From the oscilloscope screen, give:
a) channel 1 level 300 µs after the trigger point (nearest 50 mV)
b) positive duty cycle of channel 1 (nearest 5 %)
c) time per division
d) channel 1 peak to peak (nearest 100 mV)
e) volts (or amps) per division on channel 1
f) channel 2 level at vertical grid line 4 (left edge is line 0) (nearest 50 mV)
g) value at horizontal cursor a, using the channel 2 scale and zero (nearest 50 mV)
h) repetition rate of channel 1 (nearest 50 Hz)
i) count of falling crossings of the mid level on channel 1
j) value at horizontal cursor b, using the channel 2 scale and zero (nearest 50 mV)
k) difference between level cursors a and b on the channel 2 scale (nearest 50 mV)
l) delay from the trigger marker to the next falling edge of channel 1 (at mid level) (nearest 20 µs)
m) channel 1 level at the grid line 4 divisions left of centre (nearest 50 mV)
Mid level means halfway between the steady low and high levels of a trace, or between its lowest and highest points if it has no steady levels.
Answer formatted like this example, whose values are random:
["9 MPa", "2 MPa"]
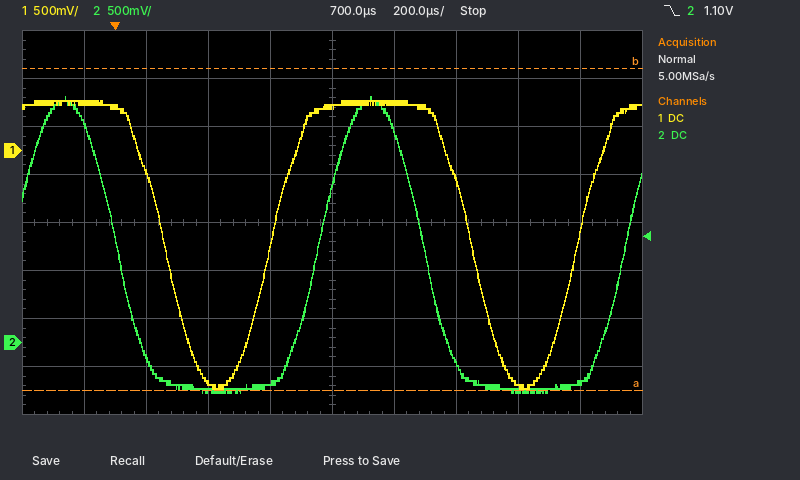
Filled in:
["-2.40 V", "65 %", "200 µs", "3.00 V", "500 mV", "-400 mV", "-500 mV", "1.00 kHz", "2", "2.85 V", "3.35 V", "160 µs", "500 mV"]
